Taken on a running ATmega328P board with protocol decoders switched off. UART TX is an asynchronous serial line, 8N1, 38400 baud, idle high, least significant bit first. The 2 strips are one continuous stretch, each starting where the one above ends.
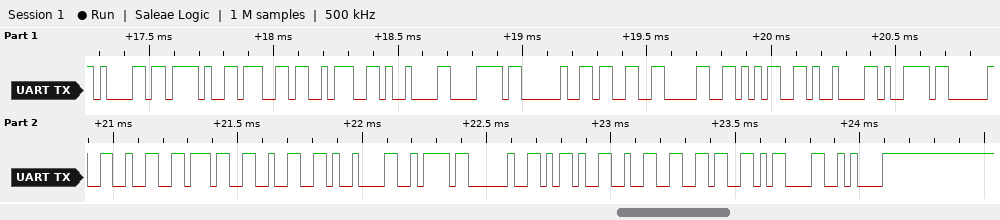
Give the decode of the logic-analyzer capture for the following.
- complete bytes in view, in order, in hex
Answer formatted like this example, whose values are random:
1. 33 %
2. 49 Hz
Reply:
1. 0x61 0x2F 0x67 0x3A 0x09 0x78 0x20 0x33 0x30 0x35 0x09 0x79 0x20 0x32 0x37 0x32 0x09 0x7A 0x20 0x2D 0x32 0x36 0x0D 0x0A
